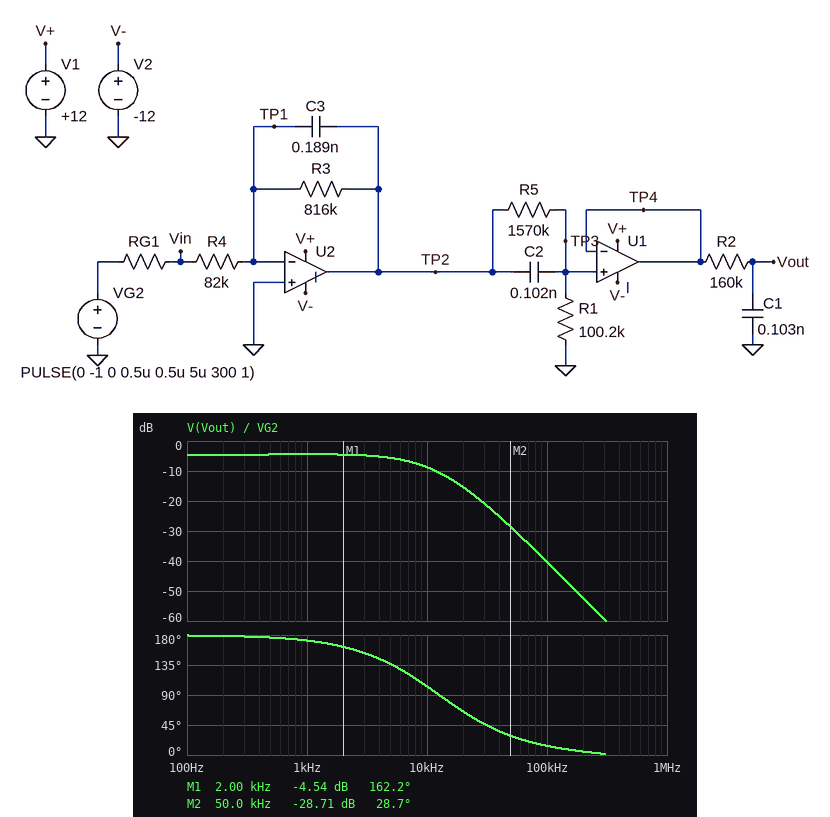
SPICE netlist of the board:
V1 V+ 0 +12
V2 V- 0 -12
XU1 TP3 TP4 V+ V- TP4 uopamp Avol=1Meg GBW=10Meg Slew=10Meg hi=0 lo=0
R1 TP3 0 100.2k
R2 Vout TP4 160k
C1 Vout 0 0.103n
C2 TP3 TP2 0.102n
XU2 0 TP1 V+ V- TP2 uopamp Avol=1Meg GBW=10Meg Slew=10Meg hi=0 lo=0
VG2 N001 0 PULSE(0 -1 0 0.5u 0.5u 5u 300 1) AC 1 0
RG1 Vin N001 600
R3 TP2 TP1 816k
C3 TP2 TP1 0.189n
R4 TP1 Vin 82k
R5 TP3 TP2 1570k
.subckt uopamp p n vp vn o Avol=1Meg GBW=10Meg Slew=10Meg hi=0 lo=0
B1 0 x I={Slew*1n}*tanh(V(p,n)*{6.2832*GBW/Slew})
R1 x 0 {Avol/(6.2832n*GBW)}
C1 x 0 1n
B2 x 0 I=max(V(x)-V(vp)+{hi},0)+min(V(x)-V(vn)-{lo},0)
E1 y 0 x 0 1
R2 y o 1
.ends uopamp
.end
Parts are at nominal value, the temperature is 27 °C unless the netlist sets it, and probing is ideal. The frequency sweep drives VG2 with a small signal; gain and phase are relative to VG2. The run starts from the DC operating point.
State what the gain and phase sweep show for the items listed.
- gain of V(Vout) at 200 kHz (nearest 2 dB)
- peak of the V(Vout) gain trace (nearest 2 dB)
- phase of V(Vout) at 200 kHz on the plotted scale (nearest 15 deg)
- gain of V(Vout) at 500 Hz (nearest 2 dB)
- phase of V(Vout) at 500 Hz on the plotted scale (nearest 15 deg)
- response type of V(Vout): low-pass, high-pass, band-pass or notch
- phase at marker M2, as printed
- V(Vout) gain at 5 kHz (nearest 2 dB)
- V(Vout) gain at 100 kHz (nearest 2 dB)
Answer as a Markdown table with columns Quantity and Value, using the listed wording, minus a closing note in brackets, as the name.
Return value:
| Quantity | Value |
|---|---|
| gain of V(Vout) at 200 kHz | -52 dB |
| peak of the V(Vout) gain trace | -4 dB |
| phase of V(Vout) at 200 kHz on the plotted scale | 0 deg |
| gain of V(Vout) at 500 Hz | -4 dB |
| phase of V(Vout) at 500 Hz on the plotted scale | 180 deg |
| response type of V(Vout): low-pass, high-pass, band-pass or notch | low-pass |
| phase at marker M2, as printed | 28.7 deg |
| V(Vout) gain at 5 kHz | -6 dB |
| V(Vout) gain at 100 kHz | -40 dB |
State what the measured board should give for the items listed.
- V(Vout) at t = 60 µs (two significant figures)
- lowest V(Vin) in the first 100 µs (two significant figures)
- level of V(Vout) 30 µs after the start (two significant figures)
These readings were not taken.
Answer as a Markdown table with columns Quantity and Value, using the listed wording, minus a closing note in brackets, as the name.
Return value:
| Quantity | Value |
|---|---|
| V(Vout) at t = 60 µs | 14 mV |
| lowest V(Vin) in the first 100 µs | -990 mV |
| level of V(Vout) 30 µs after the start | 66 mV |
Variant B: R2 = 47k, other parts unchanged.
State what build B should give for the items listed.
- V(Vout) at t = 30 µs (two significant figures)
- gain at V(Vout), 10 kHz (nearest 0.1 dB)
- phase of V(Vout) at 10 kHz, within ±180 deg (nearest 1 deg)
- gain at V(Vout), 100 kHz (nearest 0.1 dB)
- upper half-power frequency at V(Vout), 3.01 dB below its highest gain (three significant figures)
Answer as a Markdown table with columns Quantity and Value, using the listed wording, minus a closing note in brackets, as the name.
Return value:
| Quantity | Value |
|---|---|
| V(Vout) at t = 30 µs | 40 mV |
| gain at V(Vout), 10 kHz | -6.0 dB |
| phase of V(Vout) at 10 kHz, within ±180 deg | 132 deg |
| gain at V(Vout), 100 kHz | -30.1 dB |
| upper half-power frequency at V(Vout), 3.01 dB below its highest gain | 14.2 kHz |
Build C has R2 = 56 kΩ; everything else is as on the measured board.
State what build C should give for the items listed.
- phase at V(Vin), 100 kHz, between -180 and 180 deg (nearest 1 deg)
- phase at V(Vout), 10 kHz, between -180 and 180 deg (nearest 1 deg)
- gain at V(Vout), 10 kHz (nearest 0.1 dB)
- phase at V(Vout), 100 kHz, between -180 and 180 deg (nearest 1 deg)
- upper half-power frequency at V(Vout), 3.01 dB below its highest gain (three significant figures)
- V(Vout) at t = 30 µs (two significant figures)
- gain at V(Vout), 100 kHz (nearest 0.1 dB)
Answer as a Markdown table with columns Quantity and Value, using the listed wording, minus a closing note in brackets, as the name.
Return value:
| Quantity | Value |
|---|---|
| phase at V(Vin), 100 kHz, between -180 and 180 deg | 0 deg |
| phase at V(Vout), 10 kHz, between -180 and 180 deg | 129 deg |
| gain at V(Vout), 10 kHz | -6.1 dB |
| phase at V(Vout), 100 kHz, between -180 and 180 deg | 24 deg |
| upper half-power frequency at V(Vout), 3.01 dB below its highest gain | 13.5 kHz |
| V(Vout) at t = 30 µs | 45 mV |
| gain at V(Vout), 100 kHz | -31.5 dB |
